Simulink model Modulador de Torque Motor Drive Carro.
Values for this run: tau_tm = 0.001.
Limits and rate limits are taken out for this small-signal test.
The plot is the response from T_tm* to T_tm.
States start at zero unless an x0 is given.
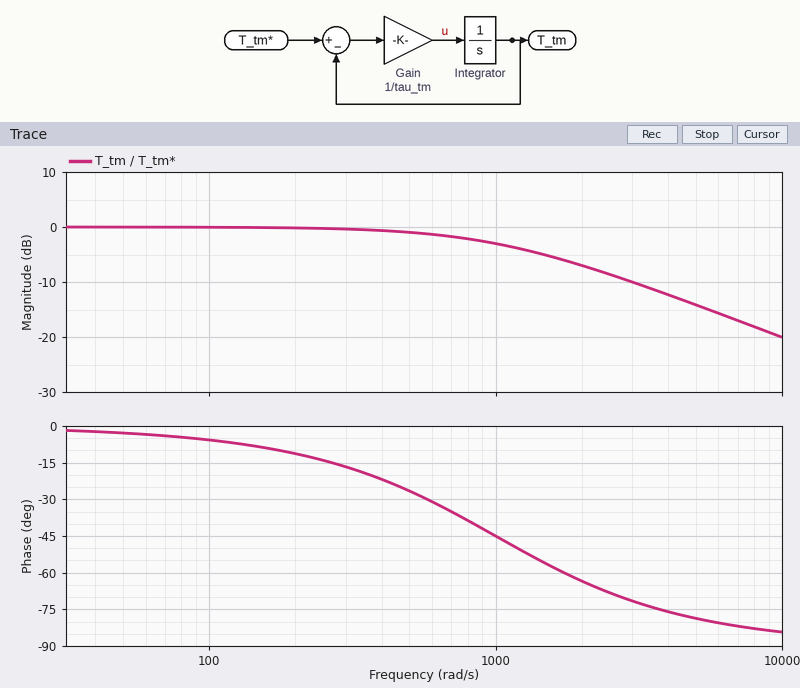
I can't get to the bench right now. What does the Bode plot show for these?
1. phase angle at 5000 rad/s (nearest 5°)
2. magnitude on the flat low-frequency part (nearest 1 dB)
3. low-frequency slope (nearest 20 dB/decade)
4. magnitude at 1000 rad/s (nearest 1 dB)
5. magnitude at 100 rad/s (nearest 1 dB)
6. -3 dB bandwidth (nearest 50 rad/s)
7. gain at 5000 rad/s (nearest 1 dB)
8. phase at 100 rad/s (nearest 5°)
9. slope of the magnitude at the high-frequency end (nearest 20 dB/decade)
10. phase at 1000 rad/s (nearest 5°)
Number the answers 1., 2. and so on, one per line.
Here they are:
1. -80°
2. 0 dB
3. 0 dB/decade
4. -3 dB
5. 0 dB
6. 1000 rad/s
7. -14 dB
8. -5°
9. -20 dB/decade
10. -45°
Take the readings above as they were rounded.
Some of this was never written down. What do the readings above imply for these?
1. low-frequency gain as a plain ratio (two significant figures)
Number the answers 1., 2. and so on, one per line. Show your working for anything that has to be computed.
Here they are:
1. 10^(0 / 20) = 1.0
